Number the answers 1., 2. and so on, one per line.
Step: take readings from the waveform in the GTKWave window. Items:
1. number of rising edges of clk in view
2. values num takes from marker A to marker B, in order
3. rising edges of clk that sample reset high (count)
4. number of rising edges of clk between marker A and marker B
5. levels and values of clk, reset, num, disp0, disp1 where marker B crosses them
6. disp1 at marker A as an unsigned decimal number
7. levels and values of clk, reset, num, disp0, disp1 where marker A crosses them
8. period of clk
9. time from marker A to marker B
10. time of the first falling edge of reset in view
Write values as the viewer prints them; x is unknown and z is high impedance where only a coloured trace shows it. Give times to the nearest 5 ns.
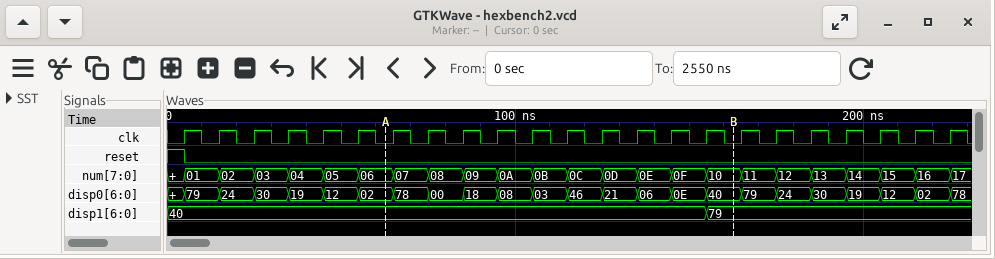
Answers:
1. 23
2. 06, 07, 08, 09, 0A, 0B, 0C, 0D, 0E, 0F, 10
3. 1
4. 10
5. clk=0, reset=0, num=10, disp0=40, disp1=79
6. 64
7. clk=0, reset=0, num=06, disp0=02, disp1=40
8. 10 ns
9. 100 ns
10. 5 ns
